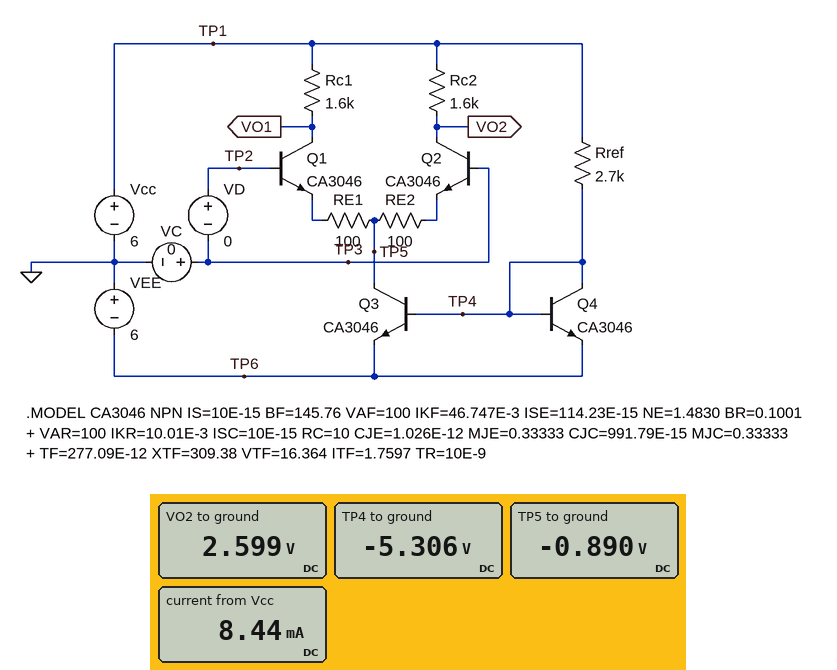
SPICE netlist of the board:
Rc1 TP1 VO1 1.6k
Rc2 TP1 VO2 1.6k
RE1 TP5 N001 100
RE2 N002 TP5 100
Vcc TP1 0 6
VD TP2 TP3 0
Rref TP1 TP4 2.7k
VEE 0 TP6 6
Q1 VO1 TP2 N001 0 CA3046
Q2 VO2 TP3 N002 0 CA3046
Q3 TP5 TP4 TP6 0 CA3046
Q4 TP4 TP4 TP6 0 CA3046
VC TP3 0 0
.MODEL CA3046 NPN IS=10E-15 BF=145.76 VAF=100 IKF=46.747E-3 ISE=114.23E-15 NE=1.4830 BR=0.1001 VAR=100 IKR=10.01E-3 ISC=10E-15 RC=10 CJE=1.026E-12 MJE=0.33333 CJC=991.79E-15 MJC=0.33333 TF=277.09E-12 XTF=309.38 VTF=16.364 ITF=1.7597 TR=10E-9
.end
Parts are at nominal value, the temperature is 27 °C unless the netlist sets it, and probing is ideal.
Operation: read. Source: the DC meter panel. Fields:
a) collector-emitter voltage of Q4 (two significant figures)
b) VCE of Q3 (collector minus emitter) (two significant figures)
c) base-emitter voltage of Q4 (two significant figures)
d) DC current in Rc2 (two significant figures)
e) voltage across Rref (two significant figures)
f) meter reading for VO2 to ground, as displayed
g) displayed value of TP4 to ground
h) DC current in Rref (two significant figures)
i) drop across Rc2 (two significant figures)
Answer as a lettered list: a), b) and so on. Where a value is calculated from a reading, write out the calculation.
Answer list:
a) -5.306 V - (-6 V) = 690 mV
b) -890 mV - (-6 V) = 5.1 V
c) -5.306 V - (-6 V) = 690 mV
d) (6 V - 2.599 V) / 1.6 kΩ = 2.1 mA
e) 6 V - (-5.306 V) = 11 V
f) 2.599 V
g) -5.306 V
h) (6 V - (-5.306 V)) / 2.7 kΩ = 4.2 mA
i) 6 V - 2.599 V = 3.4 V
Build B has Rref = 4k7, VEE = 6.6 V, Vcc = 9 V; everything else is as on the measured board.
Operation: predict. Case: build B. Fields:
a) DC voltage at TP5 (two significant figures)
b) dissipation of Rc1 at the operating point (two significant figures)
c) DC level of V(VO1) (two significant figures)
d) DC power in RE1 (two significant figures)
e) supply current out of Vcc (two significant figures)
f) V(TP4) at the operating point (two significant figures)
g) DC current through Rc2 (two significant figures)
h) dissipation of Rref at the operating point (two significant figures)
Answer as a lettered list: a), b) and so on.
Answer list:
a) -830 mV
b) 4.2 mW
c) 6.4 V
d) 270 µW
e) 6.4 mA
f) -5.9 V
g) 1.6 mA
h) 47 mW
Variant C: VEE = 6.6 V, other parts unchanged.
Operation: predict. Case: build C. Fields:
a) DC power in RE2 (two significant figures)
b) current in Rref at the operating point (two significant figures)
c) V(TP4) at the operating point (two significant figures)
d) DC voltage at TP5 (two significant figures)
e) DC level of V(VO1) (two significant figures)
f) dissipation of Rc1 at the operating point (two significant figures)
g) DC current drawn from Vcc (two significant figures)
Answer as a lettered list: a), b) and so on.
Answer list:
a) 520 µW
b) 4.4 mA
c) -5.9 V
d) -900 mV
e) 2.4 V
f) 8.1 mW
g) 8.9 mA
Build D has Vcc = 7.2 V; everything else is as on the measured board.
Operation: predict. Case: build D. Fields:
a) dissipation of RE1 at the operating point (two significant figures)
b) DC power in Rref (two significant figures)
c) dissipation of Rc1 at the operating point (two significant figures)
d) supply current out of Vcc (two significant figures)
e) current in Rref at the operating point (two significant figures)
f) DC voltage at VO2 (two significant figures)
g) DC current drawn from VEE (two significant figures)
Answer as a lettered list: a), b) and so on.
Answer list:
a) 560 µW
b) 58 mW
c) 8.8 mW
d) 9.3 mA
e) 4.6 mA
f) 3.4 V
g) 9.4 mA
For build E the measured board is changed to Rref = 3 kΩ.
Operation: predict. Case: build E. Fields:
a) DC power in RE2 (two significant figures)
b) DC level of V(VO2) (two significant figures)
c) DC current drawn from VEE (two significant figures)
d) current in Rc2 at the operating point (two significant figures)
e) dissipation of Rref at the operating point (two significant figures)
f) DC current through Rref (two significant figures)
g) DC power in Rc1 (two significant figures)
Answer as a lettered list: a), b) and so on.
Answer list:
a) 370 µW
b) 2.9 V
c) 7.6 mA
d) 1.9 mA
e) 43 mW
f) 3.8 mA
g) 5.9 mW
